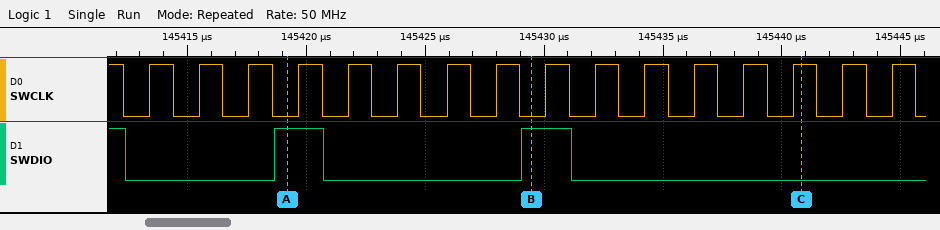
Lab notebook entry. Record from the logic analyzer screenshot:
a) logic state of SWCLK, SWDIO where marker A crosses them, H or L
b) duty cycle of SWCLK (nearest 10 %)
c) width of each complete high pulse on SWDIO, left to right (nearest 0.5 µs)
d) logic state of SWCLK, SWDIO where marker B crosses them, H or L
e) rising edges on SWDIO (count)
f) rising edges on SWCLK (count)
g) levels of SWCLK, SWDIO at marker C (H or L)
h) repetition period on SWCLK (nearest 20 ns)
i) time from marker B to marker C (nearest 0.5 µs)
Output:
SWCLK=L, SWDIO=H
50 %
2 µs, 2 µs
SWCLK=L, SWDIO=H
2
16
SWCLK=H, SWDIO=L
2080 ns
11.5 µs
